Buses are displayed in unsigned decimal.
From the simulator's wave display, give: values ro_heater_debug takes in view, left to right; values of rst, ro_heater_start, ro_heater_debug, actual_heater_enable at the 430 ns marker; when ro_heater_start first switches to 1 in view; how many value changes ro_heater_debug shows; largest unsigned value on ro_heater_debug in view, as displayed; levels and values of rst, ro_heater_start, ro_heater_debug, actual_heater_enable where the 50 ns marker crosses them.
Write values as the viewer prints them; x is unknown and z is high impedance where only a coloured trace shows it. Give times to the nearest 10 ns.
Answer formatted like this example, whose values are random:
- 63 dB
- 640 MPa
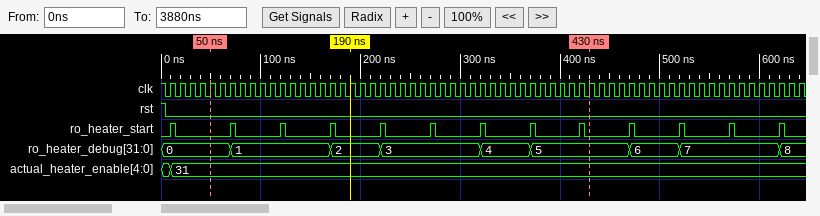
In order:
- 0, 1, 2, 3, 4, 5, 6, 7, 8
- rst=0, ro_heater_start=0, ro_heater_debug=5, actual_heater_enable=31
- 10 ns
- 8
- 8
- rst=0, ro_heater_start=0, ro_heater_debug=0, actual_heater_enable=31
